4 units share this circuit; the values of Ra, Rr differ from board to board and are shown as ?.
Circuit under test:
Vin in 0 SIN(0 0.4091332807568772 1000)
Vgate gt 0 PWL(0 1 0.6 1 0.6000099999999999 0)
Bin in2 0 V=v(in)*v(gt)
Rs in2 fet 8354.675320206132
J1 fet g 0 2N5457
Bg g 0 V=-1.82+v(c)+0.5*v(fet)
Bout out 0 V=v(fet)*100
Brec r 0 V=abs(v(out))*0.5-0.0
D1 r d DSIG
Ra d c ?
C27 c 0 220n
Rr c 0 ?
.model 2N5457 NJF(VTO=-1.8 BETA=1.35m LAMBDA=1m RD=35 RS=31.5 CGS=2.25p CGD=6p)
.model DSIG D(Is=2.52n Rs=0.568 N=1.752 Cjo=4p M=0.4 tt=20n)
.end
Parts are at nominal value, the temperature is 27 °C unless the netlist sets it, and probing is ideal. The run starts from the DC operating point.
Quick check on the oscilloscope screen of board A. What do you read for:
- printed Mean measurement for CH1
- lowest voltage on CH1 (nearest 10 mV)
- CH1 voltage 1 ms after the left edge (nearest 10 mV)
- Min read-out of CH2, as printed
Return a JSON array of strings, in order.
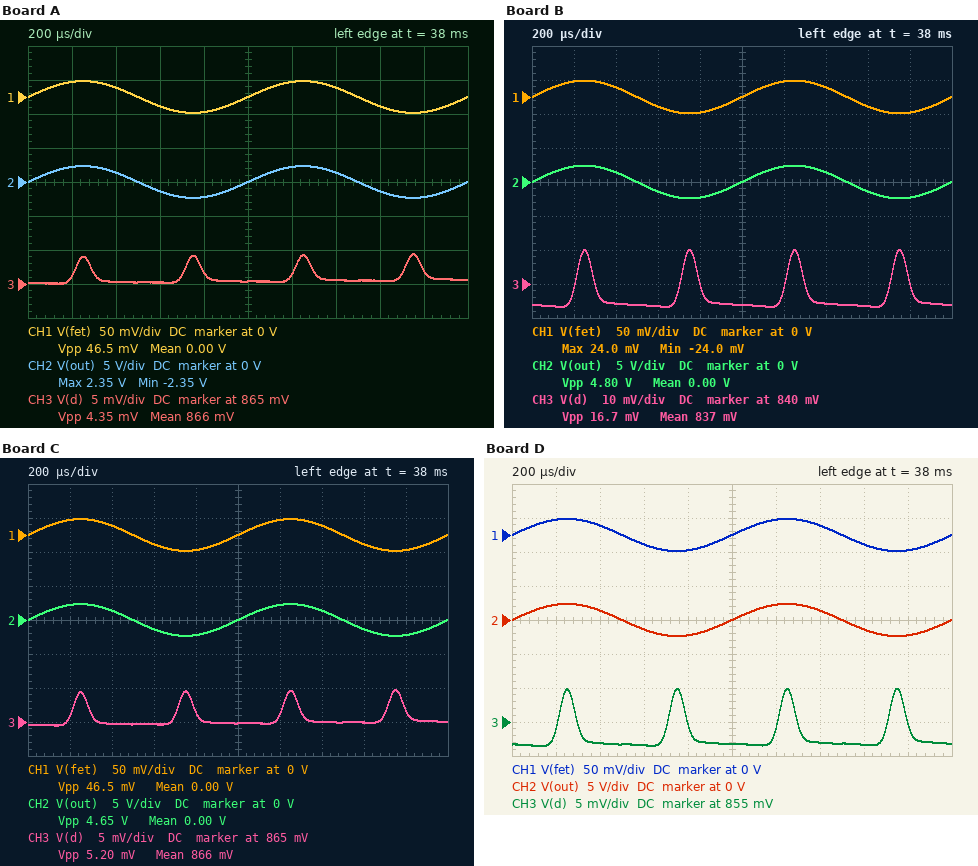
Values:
["0.00 V", "-20 mV", "0 V", "-2.35 V"]
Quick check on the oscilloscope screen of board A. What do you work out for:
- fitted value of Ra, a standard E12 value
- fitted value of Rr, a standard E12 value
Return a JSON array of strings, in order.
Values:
["2.2 kΩ", "3.9 MΩ"]
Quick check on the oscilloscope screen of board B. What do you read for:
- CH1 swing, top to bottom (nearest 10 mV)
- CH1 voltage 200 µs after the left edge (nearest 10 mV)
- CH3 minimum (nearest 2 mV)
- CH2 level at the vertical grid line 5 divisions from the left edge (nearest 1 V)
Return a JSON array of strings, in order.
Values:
["50 mV", "20 mV", "834 mV", "0 V"]
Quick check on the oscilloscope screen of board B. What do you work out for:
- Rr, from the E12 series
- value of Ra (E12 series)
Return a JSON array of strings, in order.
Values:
["820 kΩ", "2.7 kΩ"]
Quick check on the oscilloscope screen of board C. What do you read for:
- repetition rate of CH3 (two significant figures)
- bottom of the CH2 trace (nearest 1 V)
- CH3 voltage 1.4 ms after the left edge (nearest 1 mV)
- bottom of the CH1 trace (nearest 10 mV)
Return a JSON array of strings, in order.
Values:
["2.0 kHz", "-2 V", "865 mV", "-20 mV"]
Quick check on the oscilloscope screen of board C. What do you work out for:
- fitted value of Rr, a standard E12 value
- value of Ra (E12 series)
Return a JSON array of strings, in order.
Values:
["3.9 MΩ", "2.7 kΩ"]
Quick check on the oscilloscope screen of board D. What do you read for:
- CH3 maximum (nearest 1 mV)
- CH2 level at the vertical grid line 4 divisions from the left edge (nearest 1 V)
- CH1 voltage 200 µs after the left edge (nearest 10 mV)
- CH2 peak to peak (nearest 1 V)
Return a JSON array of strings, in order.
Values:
["860 mV", "-2 V", "20 mV", "5 V"]
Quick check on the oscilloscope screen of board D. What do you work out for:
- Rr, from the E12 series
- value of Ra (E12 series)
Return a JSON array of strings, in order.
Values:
["1.8 MΩ", "2.7 kΩ"]
